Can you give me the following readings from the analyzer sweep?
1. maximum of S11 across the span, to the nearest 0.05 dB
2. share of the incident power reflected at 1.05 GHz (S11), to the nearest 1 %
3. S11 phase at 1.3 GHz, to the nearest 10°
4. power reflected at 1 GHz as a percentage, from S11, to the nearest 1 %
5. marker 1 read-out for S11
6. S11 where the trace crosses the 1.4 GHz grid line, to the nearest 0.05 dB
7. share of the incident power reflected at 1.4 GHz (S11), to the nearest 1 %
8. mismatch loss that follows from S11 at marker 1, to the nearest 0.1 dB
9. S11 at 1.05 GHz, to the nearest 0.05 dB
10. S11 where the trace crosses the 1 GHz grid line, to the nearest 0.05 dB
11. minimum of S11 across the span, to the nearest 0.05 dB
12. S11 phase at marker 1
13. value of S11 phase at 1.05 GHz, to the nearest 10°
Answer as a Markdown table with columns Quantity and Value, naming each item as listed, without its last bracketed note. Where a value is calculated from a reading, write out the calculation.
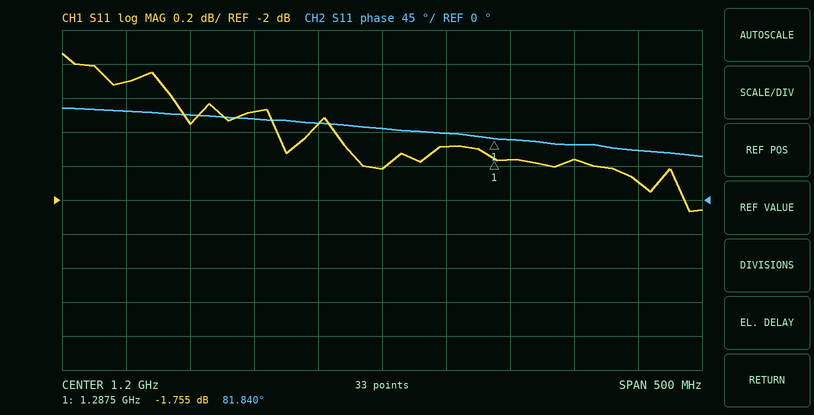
| Quantity | Value |
|---|---|
| maximum of S11 across the span, to the nearest 0.05 dB | -1.15 dB |
| share of the incident power reflected at 1.05 GHz (S11), to the nearest 1 % | 10^(-1.55/10) ≈ 70 % |
| S11 phase at 1.3 GHz, to the nearest 10° | 80° |
| power reflected at 1 GHz as a percentage, from S11, to the nearest 1 % | 10^(-1.3/10) ≈ 74 % |
| marker 1 read-out for S11 | -1.755 dB |
| S11 where the trace crosses the 1.4 GHz grid line, to the nearest 0.05 dB | -1.90 dB |
| share of the incident power reflected at 1.4 GHz (S11), to the nearest 1 % | 10^(-1.9/10) ≈ 65 % |
| mismatch loss that follows from S11 at marker 1, to the nearest 0.1 dB | −10 log10(1 − 10^(-1.755/10)) ≈ 4.8 dB |
| S11 at 1.05 GHz, to the nearest 0.05 dB | -1.55 dB |
| S11 where the trace crosses the 1 GHz grid line, to the nearest 0.05 dB | -1.30 dB |
| minimum of S11 across the span, to the nearest 0.05 dB | -2.05 dB |
| S11 phase at marker 1 | 81.840° |
| value of S11 phase at 1.05 GHz, to the nearest 10° | 110° |
